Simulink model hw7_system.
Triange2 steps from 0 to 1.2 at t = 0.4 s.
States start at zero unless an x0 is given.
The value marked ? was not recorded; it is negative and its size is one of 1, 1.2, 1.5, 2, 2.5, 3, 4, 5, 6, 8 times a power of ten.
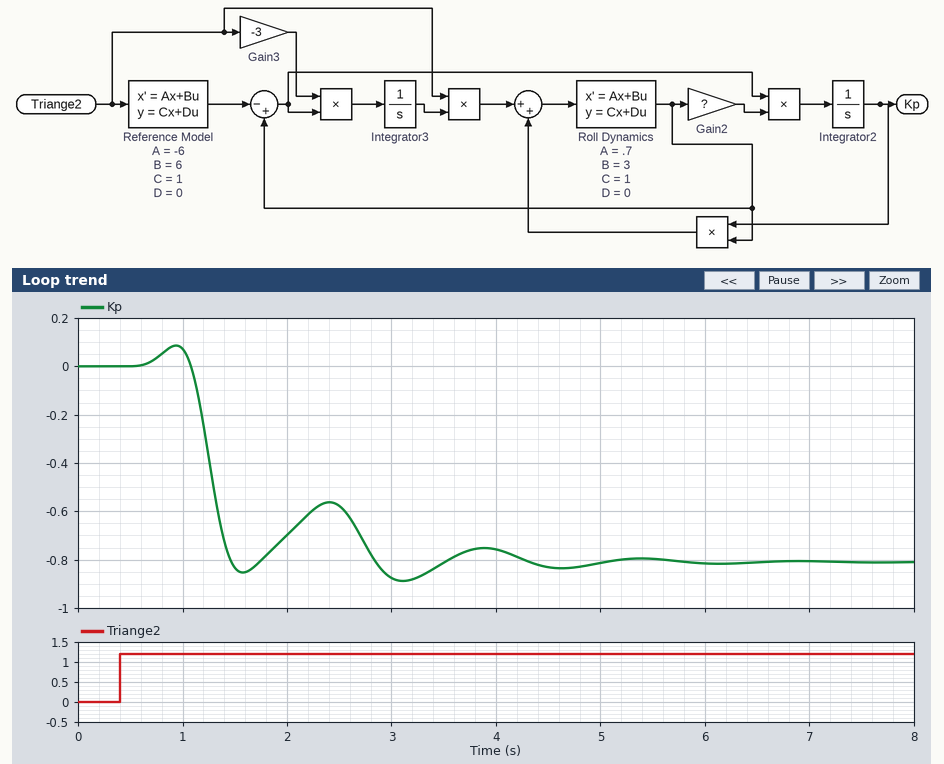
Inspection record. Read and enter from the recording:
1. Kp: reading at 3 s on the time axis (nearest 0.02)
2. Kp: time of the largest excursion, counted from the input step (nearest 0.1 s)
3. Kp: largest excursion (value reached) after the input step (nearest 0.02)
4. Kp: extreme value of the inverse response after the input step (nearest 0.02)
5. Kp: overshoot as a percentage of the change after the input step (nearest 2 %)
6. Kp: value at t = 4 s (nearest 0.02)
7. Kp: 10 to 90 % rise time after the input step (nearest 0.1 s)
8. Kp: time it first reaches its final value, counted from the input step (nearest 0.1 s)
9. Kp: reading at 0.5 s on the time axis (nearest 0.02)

-0.88
2.7 s
-0.88
0.08
10 %
-0.76
0.3 s
1.1 s
0.00
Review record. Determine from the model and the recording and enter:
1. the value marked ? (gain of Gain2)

-1.2
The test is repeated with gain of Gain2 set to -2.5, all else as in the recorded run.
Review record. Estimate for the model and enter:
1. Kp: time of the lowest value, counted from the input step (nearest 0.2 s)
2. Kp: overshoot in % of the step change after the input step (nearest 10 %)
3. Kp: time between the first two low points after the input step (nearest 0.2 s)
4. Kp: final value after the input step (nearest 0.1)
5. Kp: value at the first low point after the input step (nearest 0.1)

1.0 s
30 %
1.4 s
-0.9
-1.2
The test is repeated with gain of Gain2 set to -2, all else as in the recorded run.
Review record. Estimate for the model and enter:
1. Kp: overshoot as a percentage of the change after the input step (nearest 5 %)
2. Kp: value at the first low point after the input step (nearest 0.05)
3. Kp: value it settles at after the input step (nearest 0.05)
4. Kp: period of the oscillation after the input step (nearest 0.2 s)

20 %
-1.10
-0.90
1.4 s
